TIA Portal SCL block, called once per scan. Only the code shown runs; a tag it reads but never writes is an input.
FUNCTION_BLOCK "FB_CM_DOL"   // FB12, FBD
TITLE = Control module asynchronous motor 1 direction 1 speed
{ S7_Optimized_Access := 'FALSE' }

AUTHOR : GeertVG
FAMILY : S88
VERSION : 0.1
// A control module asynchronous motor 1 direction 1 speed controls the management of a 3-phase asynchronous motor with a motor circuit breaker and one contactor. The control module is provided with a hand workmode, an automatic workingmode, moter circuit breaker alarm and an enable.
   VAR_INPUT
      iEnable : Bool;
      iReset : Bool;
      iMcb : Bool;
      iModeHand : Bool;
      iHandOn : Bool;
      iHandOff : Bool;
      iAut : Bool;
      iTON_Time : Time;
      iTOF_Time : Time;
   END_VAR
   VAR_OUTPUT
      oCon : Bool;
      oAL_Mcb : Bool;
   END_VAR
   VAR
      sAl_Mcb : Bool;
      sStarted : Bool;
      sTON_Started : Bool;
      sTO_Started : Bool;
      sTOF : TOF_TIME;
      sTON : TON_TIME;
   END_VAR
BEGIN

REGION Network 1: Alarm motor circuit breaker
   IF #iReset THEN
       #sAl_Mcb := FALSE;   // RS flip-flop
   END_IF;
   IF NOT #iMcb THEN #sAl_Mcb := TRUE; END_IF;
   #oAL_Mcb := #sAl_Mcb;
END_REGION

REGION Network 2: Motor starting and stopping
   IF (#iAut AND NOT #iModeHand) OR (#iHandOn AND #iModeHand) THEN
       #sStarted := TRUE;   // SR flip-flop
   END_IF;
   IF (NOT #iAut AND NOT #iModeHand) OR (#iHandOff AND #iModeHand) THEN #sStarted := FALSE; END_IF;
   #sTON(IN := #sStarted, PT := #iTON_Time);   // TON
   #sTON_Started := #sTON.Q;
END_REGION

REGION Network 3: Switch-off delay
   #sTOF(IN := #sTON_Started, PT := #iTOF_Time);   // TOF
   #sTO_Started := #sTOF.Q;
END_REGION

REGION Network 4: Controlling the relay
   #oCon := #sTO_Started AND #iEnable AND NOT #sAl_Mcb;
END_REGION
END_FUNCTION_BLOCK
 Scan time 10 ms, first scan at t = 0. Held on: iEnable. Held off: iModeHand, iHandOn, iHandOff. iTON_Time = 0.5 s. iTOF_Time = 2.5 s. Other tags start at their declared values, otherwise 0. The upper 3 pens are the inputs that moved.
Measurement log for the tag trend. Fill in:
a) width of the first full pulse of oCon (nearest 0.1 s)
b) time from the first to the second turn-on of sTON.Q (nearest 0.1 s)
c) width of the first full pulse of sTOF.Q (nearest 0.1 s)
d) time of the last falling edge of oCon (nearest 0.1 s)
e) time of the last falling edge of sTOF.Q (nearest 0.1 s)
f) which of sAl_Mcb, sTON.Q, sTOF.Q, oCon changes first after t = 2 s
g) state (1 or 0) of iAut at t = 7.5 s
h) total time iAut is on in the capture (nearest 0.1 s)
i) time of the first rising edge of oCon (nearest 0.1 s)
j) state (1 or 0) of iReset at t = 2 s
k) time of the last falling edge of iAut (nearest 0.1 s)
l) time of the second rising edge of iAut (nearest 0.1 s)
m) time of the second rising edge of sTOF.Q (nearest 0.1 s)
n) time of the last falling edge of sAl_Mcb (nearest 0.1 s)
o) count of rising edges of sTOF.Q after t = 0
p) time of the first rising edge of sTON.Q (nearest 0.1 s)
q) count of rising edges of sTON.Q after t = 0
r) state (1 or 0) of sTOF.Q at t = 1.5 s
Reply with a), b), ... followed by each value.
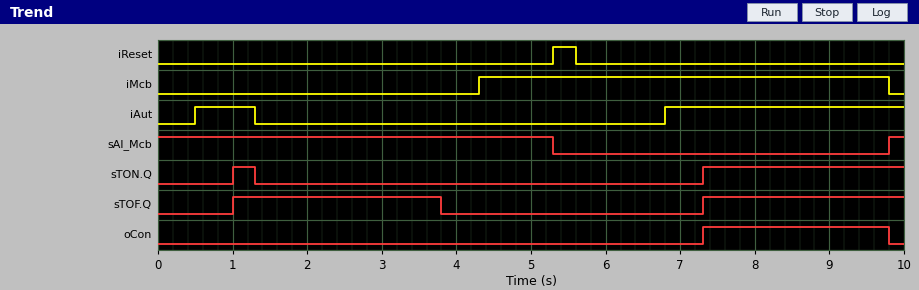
a) 2.5 s
b) 6.3 s
c) 2.8 s
d) 9.8 s
e) 3.8 s
f) sTOF.Q
g) 1
h) 4.0 s
i) 7.3 s
j) 0
k) 1.3 s
l) 6.8 s
m) 7.3 s
n) 5.3 s
o) 2
p) 1.0 s
q) 2
r) 1
